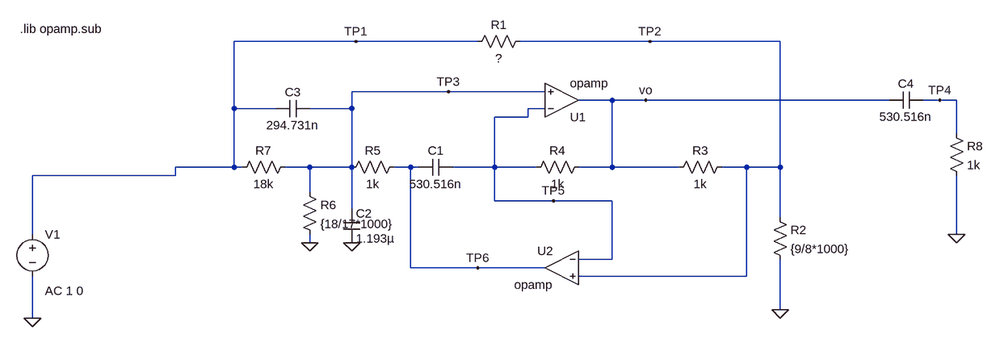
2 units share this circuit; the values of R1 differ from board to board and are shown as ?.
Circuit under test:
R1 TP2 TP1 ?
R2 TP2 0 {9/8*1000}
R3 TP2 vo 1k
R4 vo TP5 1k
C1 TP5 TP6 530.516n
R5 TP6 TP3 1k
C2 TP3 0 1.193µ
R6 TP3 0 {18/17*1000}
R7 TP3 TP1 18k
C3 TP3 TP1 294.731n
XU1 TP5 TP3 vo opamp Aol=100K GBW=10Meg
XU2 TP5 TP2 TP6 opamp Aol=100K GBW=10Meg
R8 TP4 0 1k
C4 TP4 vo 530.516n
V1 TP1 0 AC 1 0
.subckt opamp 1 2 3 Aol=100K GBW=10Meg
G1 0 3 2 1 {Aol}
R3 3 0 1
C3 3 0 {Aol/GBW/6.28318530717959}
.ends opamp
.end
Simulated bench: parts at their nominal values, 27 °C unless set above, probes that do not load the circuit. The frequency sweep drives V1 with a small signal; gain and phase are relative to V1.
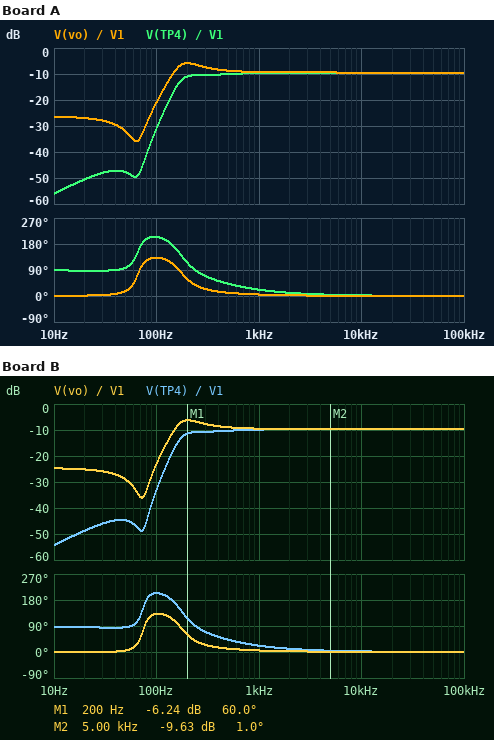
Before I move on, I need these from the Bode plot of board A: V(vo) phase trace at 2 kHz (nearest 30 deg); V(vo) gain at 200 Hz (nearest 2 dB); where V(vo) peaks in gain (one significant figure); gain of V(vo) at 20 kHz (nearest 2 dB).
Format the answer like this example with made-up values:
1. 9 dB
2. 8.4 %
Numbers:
1. 0 deg
2. -6 dB
3. 200 Hz
4. -10 dB
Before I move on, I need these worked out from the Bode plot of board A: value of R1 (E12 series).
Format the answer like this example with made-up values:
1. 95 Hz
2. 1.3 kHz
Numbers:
1. 22 kΩ
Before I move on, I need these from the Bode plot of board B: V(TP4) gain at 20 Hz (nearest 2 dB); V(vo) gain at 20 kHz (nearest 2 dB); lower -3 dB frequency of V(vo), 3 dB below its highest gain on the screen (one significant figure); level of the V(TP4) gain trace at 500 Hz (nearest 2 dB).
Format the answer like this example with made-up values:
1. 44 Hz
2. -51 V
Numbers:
1. -48 dB
2. -10 dB
3. 200 Hz
4. -10 dB
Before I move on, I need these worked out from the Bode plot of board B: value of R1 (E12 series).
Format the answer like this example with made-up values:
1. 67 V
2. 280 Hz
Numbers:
1. 18 kΩ
